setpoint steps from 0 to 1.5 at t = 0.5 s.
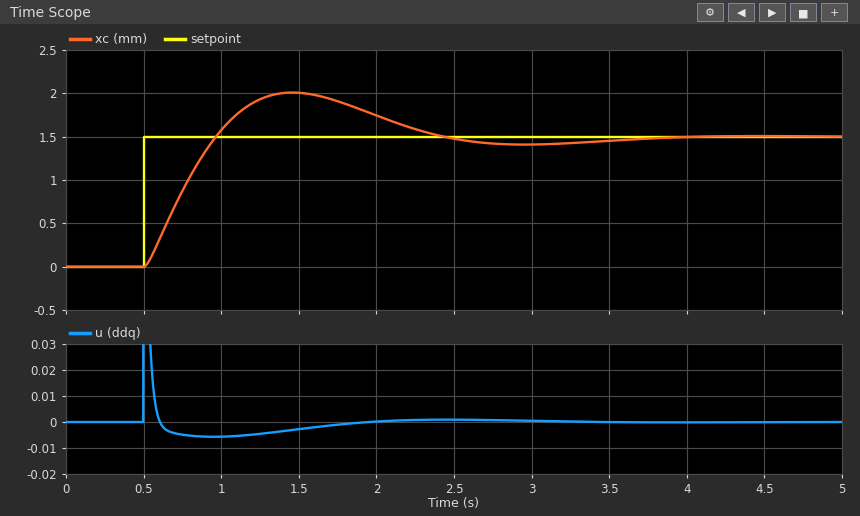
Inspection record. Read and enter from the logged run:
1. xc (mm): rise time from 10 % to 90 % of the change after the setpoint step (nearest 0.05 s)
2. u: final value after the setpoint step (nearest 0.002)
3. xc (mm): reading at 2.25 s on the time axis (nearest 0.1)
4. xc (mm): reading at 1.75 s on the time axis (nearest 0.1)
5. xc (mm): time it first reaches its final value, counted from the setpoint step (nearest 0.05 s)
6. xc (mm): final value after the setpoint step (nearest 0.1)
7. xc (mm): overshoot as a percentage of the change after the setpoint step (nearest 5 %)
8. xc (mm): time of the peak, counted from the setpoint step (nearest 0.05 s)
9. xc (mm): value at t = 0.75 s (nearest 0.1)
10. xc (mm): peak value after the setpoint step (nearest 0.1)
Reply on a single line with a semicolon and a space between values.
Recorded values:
0.35 s; 0.000; 1.6; 1.9; 0.45 s; 1.5; 35 %; 0.95 s; 0.9; 2.0
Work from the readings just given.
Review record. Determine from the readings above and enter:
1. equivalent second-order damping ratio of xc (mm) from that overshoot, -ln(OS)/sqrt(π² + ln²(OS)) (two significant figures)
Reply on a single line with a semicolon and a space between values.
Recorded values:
0.32
